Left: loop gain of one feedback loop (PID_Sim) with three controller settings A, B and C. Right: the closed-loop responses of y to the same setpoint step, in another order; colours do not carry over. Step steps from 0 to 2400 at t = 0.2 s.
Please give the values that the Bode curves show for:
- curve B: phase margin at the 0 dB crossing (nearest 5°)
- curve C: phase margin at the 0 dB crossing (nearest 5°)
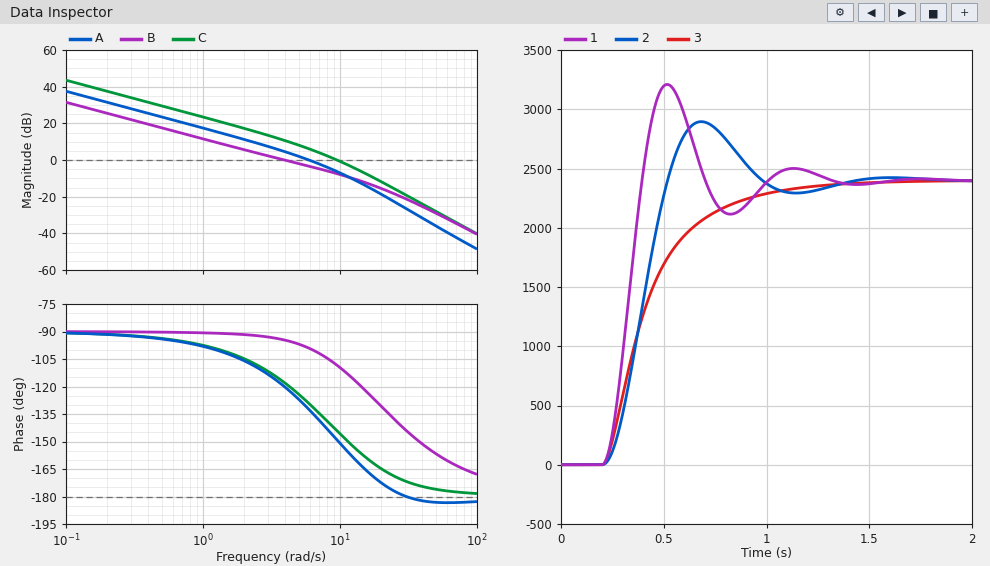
85°
35°
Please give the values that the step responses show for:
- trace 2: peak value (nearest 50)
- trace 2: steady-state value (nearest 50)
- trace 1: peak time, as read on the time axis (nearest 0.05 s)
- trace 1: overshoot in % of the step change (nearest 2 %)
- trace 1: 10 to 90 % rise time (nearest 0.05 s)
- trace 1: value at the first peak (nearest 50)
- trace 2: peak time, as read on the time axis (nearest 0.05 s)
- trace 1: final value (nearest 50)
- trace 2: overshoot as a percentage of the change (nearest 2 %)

2900
2400
0.50 s
34 %
0.15 s
3200
0.70 s
2400
20 %
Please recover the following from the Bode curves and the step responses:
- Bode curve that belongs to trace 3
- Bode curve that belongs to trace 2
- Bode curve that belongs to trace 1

B
A
C
